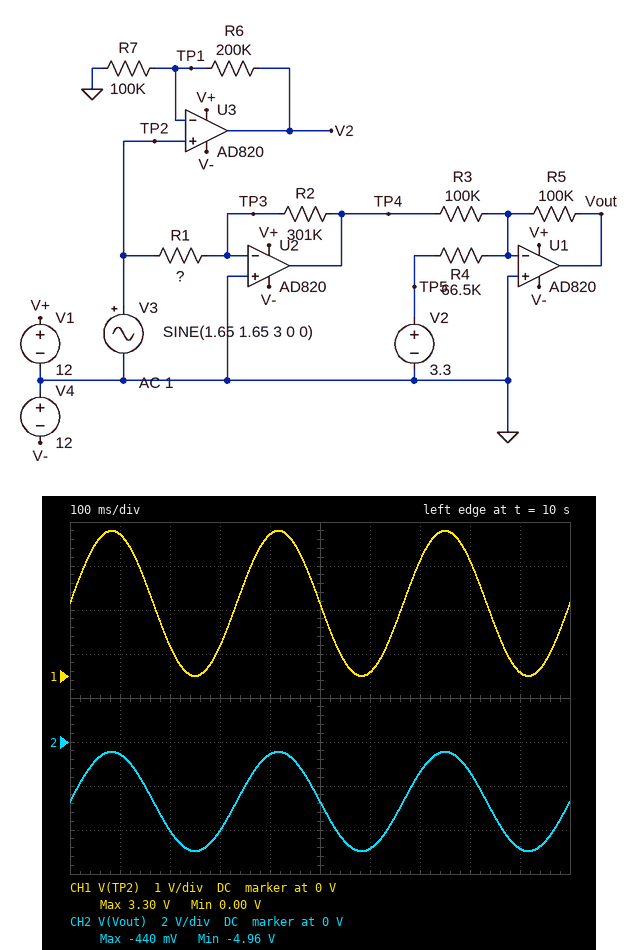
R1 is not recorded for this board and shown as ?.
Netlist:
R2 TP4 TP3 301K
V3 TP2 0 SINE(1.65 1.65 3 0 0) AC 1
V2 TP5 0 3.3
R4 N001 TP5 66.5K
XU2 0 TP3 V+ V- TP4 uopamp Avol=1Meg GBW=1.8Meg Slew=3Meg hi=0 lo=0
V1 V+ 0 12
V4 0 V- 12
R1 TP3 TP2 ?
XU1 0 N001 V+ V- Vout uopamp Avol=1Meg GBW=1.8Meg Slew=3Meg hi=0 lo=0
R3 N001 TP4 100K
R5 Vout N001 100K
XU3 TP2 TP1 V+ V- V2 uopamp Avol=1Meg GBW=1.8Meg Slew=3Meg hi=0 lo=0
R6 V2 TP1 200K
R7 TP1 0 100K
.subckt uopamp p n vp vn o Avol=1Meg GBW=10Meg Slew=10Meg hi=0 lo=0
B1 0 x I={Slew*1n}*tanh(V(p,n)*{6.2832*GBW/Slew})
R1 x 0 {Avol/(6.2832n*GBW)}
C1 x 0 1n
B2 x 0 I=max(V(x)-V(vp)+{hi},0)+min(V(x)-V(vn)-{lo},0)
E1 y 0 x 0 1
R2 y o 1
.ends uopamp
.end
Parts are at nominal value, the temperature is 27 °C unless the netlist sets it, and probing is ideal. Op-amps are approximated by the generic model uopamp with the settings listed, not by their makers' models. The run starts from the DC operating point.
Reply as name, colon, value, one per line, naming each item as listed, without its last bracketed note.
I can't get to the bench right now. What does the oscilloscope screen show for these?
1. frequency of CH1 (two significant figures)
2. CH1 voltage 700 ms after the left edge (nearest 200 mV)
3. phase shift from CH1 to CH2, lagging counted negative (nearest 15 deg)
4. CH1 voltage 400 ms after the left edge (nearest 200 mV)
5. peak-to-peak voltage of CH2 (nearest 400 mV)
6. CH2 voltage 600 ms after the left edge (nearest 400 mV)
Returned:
frequency of CH1: 3.0 Hz
CH1 voltage 700 ms after the left edge: 2.6 V
phase shift from CH1 to CH2, lagging counted negative: 0 deg
CH1 voltage 400 ms after the left edge: 3.2 V
peak-to-peak voltage of CH2: 4.4 V
CH2 voltage 600 ms after the left edge: -4.8 V
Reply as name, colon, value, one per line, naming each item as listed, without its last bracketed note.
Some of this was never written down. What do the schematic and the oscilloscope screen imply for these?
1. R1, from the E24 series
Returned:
R1, from the E24 series: 220 kΩ
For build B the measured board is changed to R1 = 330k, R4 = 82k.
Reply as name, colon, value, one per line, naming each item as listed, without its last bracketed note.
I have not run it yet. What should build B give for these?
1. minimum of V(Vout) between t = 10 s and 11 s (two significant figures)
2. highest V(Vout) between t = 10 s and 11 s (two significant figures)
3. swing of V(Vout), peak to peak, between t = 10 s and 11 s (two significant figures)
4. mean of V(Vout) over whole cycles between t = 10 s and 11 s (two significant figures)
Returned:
minimum of V(Vout) between t = 10 s and 11 s: -4.0 V
highest V(Vout) between t = 10 s and 11 s: -1.0 V
swing of V(Vout), peak to peak, between t = 10 s and 11 s: 3.0 V
mean of V(Vout) over whole cycles between t = 10 s and 11 s: -2.5 V
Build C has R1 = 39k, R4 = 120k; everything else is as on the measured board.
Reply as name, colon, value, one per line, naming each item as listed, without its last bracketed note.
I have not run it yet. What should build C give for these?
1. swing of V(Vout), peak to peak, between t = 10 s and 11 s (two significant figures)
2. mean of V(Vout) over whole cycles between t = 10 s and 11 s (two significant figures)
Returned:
swing of V(Vout), peak to peak, between t = 10 s and 11 s: 12 V
mean of V(Vout) over whole cycles between t = 10 s and 11 s: 5.6 V
